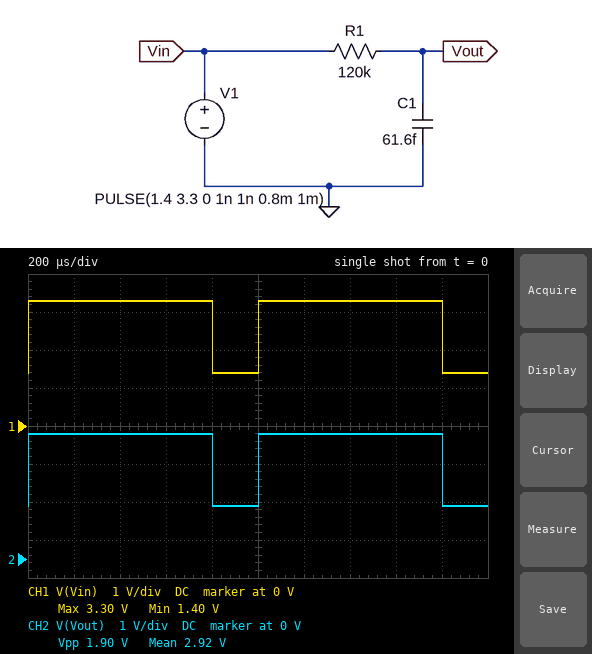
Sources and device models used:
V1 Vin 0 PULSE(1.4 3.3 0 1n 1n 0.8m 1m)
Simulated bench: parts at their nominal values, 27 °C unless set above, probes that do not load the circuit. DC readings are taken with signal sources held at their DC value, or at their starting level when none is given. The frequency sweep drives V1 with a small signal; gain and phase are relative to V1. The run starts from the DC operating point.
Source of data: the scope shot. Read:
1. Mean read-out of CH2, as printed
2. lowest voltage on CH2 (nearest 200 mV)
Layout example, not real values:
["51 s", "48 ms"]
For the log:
["2.92 V", "1.4 V"]
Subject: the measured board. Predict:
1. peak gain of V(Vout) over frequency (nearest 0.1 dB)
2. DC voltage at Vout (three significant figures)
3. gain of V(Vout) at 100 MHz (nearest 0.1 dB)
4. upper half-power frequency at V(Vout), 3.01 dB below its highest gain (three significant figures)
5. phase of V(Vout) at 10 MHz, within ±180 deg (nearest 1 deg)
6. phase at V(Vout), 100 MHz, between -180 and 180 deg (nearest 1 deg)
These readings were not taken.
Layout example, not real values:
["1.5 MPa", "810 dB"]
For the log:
["0 dB", "1.40 V", "-13.5 dB", "21.5 MHz", "-25 deg", "-78 deg"]
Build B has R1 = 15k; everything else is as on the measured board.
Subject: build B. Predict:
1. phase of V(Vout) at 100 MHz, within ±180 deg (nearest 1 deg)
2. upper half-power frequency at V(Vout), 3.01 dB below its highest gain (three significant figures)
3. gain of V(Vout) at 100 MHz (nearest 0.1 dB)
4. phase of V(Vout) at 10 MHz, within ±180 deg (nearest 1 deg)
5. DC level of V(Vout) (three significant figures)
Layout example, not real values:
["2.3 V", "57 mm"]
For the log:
["-30 deg", "172 MHz", "-1.3 dB", "-3 deg", "1.40 V"]
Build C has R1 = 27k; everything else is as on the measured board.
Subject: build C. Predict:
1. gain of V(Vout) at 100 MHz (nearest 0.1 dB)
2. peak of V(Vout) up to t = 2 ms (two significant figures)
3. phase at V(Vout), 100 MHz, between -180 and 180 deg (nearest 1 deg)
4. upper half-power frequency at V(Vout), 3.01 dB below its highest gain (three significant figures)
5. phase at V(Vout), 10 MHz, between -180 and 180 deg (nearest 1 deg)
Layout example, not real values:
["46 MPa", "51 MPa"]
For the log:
["-3.2 dB", "3.3 V", "-46 deg", "95.7 MHz", "-6 deg"]
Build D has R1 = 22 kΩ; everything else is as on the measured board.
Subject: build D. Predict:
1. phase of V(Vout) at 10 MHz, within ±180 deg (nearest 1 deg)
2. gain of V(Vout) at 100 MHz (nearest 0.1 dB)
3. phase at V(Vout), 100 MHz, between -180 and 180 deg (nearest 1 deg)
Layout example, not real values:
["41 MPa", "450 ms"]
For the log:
["-5 deg", "-2.4 dB", "-40 deg"]
